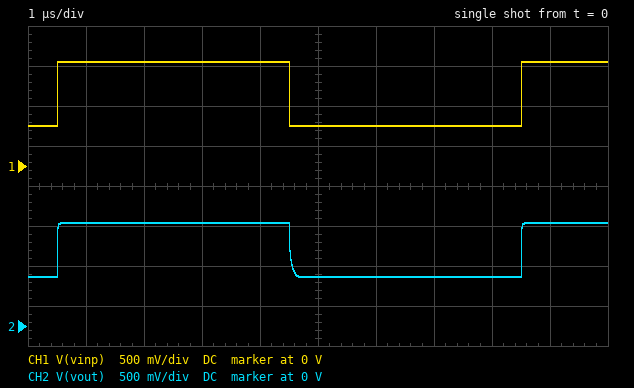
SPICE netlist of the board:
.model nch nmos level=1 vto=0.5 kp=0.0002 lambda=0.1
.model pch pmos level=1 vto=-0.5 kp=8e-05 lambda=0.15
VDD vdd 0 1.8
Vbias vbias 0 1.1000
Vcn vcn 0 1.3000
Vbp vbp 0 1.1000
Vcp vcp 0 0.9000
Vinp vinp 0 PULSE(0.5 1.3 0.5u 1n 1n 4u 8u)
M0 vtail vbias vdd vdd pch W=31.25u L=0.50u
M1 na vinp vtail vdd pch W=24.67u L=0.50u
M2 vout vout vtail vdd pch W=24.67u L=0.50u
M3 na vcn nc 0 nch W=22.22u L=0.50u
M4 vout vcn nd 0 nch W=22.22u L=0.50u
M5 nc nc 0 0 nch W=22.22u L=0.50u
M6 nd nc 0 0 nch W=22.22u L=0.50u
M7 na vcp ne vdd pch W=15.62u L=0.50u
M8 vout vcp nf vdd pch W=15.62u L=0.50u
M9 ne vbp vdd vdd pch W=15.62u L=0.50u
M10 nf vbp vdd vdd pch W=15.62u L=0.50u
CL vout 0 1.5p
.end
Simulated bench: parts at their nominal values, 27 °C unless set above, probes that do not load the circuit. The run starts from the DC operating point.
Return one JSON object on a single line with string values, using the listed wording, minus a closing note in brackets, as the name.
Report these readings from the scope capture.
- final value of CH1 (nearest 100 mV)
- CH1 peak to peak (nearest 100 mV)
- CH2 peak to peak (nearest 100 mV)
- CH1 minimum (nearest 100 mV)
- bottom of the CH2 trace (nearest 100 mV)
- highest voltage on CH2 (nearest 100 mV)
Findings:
{"final value of CH1": "1.3 V", "CH1 peak to peak": "800 mV", "CH2 peak to peak": "700 mV", "CH1 minimum": "500 mV", "bottom of the CH2 trace": "600 mV", "highest voltage on CH2": "1.3 V"}
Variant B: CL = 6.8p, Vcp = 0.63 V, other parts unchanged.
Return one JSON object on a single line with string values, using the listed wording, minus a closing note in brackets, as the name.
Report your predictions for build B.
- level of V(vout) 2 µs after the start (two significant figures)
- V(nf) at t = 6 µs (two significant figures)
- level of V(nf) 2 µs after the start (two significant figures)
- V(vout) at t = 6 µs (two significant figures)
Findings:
{"level of V(vout) 2 µs after the start": "1.3 V", "V(nf) at t = 6 µs": "1.3 V", "level of V(nf) 2 µs after the start": "1.4 V", "V(vout) at t = 6 µs": "710 mV"}
